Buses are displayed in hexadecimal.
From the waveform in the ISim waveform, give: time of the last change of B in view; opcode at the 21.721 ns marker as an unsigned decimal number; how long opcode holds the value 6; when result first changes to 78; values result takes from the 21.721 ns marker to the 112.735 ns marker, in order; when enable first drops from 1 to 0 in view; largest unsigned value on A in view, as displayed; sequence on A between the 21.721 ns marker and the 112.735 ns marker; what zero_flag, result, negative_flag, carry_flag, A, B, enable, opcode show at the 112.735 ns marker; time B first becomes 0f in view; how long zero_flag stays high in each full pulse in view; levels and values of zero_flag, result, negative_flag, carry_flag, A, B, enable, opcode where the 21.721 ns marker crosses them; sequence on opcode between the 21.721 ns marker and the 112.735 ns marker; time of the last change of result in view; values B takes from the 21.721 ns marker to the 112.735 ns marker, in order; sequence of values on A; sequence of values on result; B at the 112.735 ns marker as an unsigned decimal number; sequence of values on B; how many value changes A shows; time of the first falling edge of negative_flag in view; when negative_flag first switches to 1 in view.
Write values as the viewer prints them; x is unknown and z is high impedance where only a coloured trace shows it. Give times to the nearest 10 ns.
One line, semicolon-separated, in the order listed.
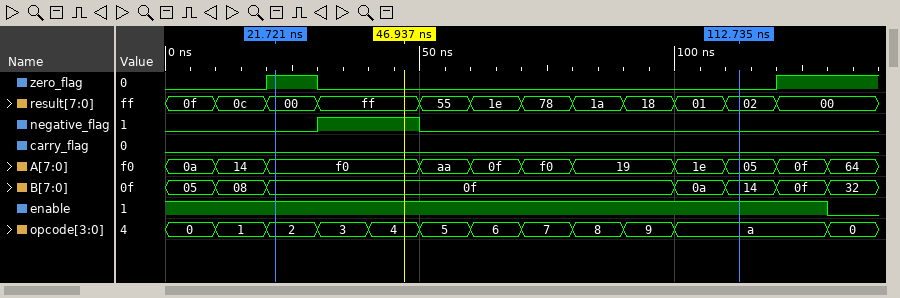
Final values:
130 ns; 2; 10 ns; 70 ns; 00, ff, 55, 1e, 78, 1a, 18, 01, 02; 130 ns; f0; f0, aa, 0f, f0, 19, 1e, 05; zero_flag=0, result=02, negative_flag=0, carry_flag=0, A=05, B=14, enable=1, opcode=a; 20 ns; 10 ns; zero_flag=1, result=00, negative_flag=0, carry_flag=0, A=f0, B=0f, enable=1, opcode=2; 2, 3, 4, 5, 6, 7, 8, 9, a; 120 ns; 0f, 0a, 14; 0a, 14, f0, aa, 0f, f0, 19, 1e, 05, 0f, 64; 0f, 0c, 00, ff, 55, 1e, 78, 1a, 18, 01, 02, 00; 20; 05, 08, 0f, 0a, 14, 0f, 32; 10; 50 ns; 30 ns
